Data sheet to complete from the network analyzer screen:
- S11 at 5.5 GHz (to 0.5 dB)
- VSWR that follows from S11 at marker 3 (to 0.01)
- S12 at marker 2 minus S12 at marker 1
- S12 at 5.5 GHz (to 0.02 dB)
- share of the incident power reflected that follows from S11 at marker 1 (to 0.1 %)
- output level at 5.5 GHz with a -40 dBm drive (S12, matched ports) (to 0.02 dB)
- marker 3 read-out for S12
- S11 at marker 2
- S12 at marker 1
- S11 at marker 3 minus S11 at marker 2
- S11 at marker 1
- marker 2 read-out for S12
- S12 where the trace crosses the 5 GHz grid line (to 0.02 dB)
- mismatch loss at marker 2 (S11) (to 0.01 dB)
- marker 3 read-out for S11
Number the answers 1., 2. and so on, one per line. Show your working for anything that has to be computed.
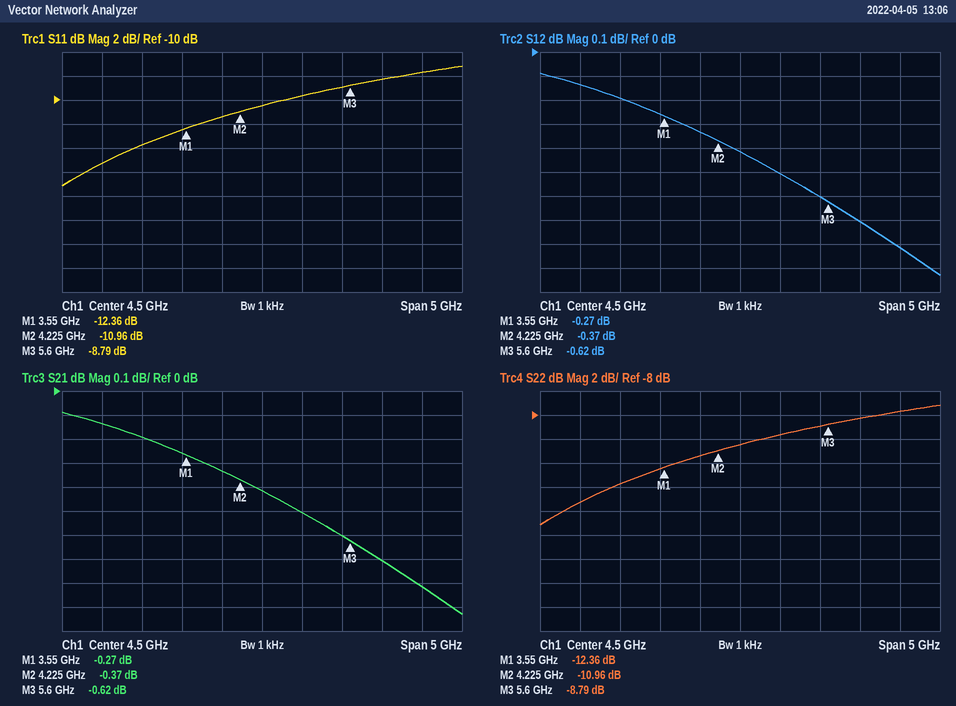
1. -9.0 dB
2. (1 + 0.3635)/(1 − 0.3635) ≈ 2.14
3. -0.37 − (-0.27) = -0.10 dB
4. -0.60 dB
5. 10^(-12.36/10) ≈ 5.8 %
6. -40 dBm + (-0.60 dB) = -40.60 dBm
7. -0.62 dB
8. -10.96 dB
9. -0.27 dB
10. -8.79 − (-10.96) = 2.17 dB
11. -12.36 dB
12. -0.37 dB
13. -0.50 dB
14. −10 log10(1 − 10^(-10.96/10)) ≈ 0.36 dB
15. -8.79 dB
